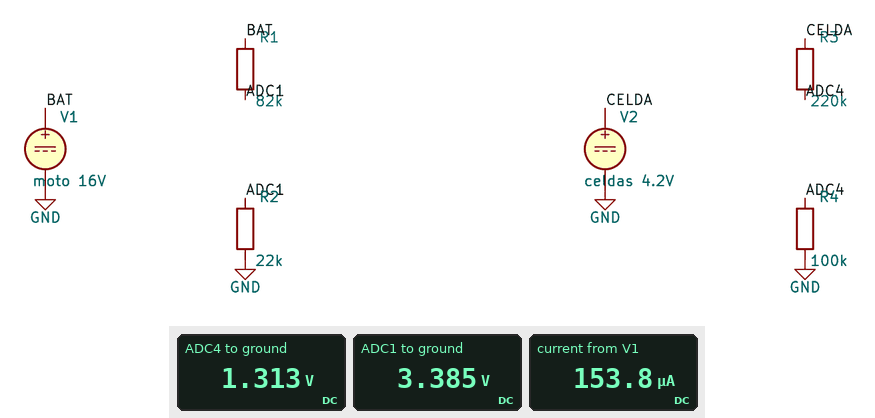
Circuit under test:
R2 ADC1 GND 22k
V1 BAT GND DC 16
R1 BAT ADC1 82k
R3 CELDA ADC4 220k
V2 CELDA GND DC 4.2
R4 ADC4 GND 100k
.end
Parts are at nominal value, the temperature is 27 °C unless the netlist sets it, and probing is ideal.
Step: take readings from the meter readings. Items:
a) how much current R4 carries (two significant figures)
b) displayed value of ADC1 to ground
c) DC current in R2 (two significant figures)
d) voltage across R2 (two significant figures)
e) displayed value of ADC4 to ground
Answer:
13 µA
3.385 V
150 µA
3.4 V
1.313 V
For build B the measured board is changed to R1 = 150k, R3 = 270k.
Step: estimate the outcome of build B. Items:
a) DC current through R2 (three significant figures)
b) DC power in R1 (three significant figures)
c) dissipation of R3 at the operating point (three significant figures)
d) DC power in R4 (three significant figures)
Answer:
93.0 µA
1.30 mW
34.8 µW
12.9 µW
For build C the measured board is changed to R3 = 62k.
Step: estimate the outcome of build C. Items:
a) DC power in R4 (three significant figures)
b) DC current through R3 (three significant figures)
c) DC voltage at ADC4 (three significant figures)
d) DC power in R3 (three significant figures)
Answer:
67.2 µW
25.9 µA
2.59 V
41.7 µW
